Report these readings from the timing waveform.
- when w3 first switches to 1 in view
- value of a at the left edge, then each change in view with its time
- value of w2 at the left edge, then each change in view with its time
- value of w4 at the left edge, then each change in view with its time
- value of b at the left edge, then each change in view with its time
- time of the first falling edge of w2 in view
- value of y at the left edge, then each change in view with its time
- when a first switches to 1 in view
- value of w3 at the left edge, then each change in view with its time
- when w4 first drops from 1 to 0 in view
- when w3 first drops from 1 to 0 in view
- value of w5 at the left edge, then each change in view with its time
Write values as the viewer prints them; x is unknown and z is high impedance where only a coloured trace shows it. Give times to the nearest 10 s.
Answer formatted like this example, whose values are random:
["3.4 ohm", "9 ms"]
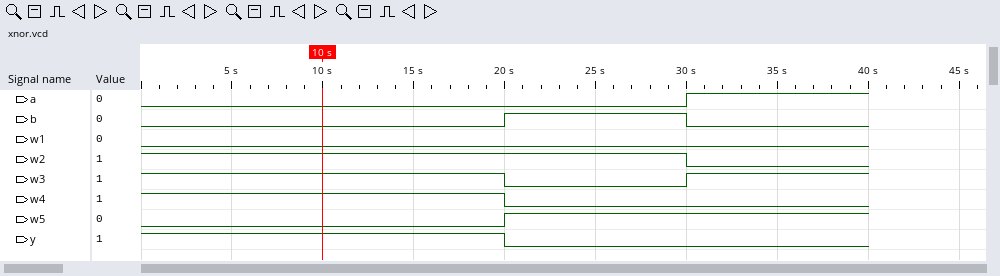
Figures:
["30 s", "0, 1 at 30 s", "1, 0 at 30 s", "1, 0 at 20 s", "0, 1 at 20 s, 0 at 30 s", "30 s", "1, 0 at 20 s", "30 s", "1, 0 at 20 s, 1 at 30 s", "20 s", "20 s", "0, 1 at 20 s"]
